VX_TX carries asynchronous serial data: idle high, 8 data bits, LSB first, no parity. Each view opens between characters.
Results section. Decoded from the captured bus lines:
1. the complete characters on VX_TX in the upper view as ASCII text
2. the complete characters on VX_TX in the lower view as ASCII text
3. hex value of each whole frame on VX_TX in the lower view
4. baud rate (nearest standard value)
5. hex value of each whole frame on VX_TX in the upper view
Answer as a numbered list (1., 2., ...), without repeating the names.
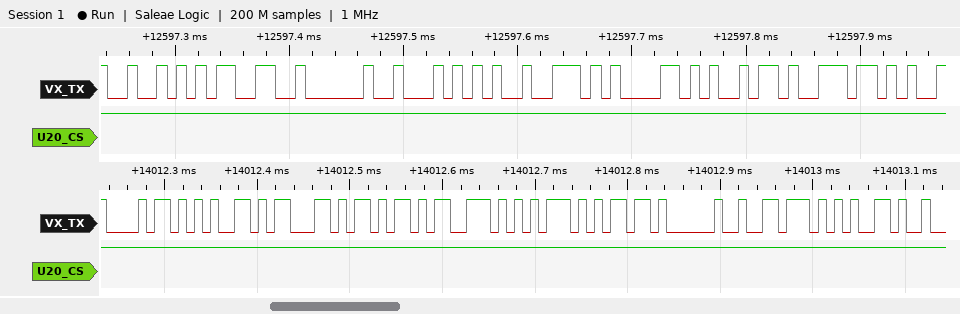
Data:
1. "R3 Train"
2. "hecksum ve"
3. 68, 65, 63, 6B, 73, 75, 6D, 20, 76, 65
4. 115200 baud
5. 52, 33, 20, 54, 72, 61, 69, 6E
